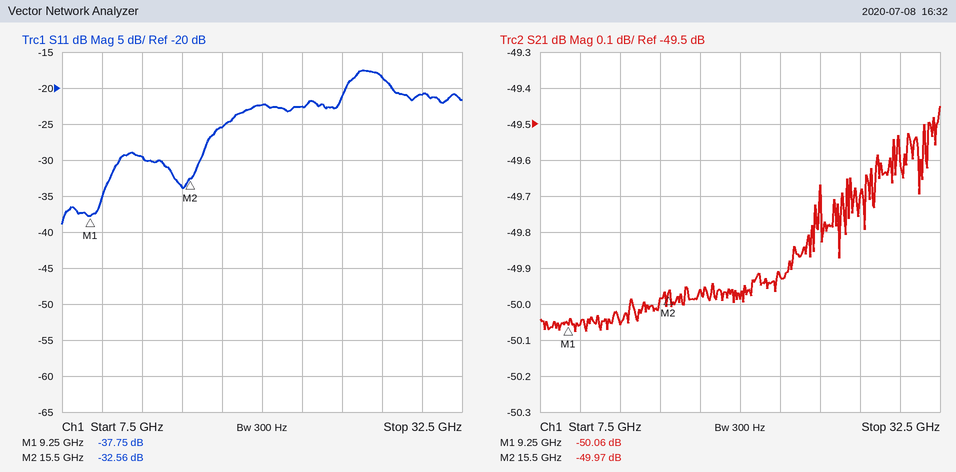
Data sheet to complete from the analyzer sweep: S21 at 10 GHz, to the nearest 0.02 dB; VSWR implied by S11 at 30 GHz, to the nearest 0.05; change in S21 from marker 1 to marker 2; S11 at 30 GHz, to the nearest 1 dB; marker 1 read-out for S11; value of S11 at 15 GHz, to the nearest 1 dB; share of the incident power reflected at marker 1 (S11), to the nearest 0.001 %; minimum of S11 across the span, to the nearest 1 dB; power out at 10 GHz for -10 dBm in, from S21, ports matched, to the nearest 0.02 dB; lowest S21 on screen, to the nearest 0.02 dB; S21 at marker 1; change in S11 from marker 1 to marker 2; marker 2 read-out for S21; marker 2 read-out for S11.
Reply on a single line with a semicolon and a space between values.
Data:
-50.06 dB; 1.20; 0.09 dB; -21 dB; -37.75 dB; -34 dB; 0.017 %; -39 dB; -60.06 dBm; -50.08 dB; -50.06 dB; 5.19 dB; -49.97 dB; -32.56 dB
